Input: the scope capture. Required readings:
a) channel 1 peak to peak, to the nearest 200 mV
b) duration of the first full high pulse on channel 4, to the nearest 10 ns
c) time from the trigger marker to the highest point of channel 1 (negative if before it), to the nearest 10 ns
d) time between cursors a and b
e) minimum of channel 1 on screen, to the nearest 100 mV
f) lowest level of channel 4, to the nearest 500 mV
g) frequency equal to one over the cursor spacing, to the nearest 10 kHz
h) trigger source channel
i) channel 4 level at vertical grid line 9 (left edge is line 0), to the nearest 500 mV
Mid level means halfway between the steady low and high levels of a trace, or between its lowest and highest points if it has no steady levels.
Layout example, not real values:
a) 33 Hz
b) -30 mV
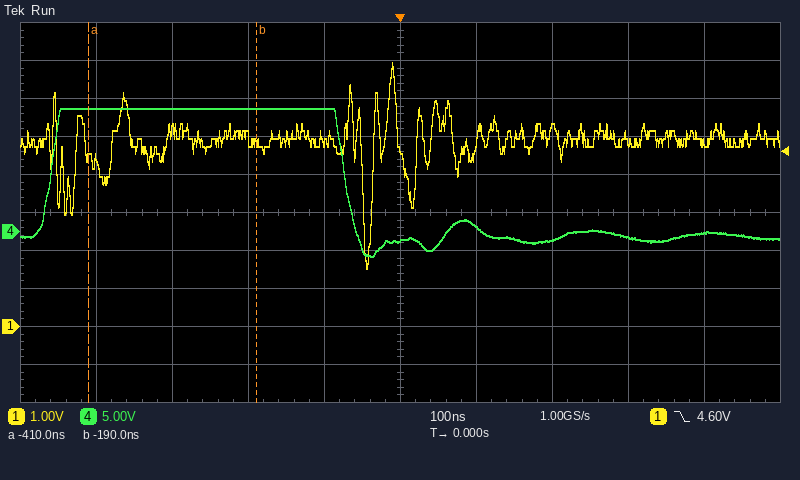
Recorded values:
a) 5.4 V
b) 390 ns
c) -10 ns
d) 220 ns
e) 1.5 V
f) -3.5 V
g) 4.55 MHz
h) channel 1
i) 0.0 V
